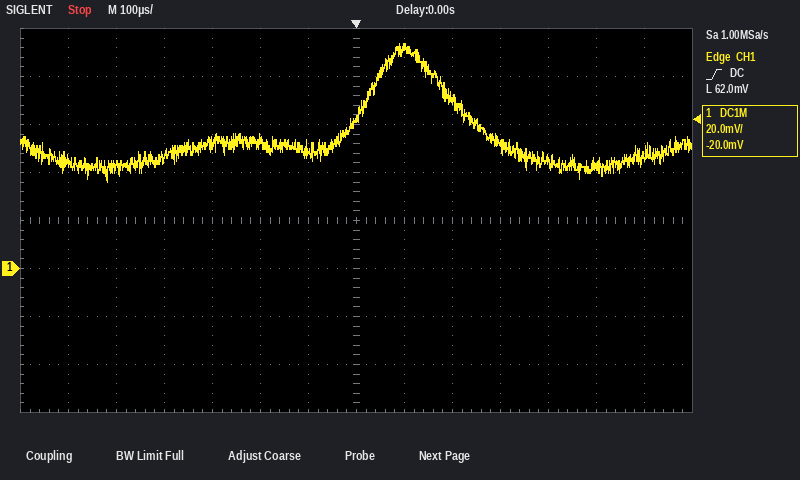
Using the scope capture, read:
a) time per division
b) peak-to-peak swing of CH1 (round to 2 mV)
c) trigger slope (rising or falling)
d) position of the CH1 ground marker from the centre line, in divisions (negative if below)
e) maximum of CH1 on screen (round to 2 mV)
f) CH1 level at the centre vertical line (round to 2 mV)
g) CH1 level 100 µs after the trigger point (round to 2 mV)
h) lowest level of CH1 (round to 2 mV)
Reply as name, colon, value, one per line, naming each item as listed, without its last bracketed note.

time per division: 100 µs
peak-to-peak swing of CH1: 58 mV
trigger slope: rising
position of the CH1 ground marker from the centre line, in divisions: -1.0 div
maximum of CH1 on screen: 94 mV
CH1 level at the centre vertical line: 62 mV
CH1 level 100 µs after the trigger point: 92 mV
lowest level of CH1: 36 mV
